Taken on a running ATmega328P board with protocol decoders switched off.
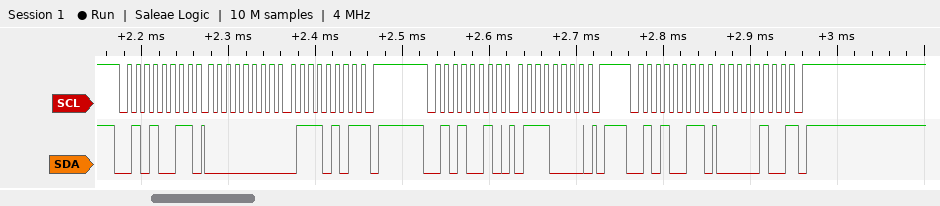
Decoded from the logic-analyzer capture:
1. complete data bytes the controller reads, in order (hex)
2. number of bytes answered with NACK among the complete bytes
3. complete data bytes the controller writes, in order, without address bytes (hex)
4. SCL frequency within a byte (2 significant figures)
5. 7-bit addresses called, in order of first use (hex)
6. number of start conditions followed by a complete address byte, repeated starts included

00 75 04
2
70
100 kHz
0x29
3
